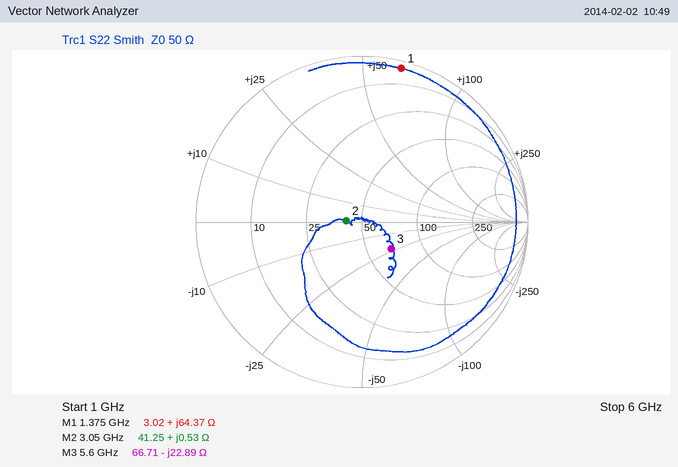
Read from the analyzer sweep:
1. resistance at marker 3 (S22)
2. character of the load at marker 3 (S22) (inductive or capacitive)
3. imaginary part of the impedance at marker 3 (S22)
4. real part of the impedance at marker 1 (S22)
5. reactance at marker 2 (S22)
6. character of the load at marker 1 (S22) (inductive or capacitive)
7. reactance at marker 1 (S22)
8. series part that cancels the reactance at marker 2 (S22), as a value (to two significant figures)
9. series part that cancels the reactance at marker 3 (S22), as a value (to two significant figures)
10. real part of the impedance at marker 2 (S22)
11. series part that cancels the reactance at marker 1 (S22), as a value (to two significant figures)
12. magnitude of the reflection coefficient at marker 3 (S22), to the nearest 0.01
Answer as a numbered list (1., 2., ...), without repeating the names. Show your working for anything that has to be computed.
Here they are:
1. 66.71 Ω
2. capacitive
3. -22.89 Ω
4. 3.02 Ω
5. +0.53 Ω
6. inductive
7. +64.37 Ω
8. C = 1/(2π × 3.05 GHz × 0.53 Ω) ≈ 98 pF
9. L = 22.89 Ω/(2π × 5.6 GHz) ≈ 651 pH, so 650 pH to two significant figures
10. 41.25 Ω
11. C = 1/(2π × 1.375 GHz × 64.37 Ω) ≈ 1.8 pF
12. 0.24
